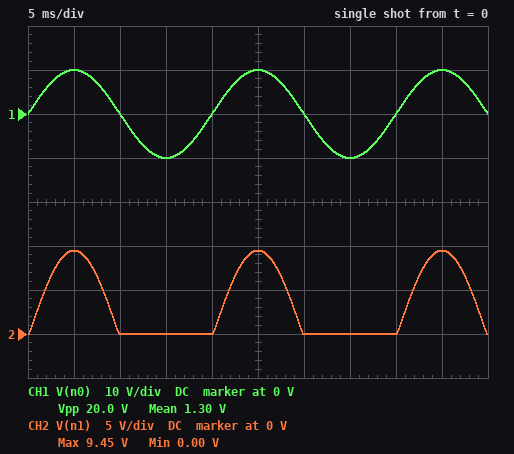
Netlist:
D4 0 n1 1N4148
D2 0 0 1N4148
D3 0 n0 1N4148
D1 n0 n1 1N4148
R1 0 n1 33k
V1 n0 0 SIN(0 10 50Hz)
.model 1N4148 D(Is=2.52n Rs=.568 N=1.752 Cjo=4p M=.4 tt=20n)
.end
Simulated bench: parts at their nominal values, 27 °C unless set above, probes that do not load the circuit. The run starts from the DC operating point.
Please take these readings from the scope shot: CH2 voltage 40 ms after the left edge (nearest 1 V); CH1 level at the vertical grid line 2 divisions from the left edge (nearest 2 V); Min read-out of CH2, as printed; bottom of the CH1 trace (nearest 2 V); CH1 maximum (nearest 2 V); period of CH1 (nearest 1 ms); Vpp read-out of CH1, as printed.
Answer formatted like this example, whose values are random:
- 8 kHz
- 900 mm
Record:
- 0 V
- 0 V
- 0.00 V
- -10 V
- 10 V
- 20 ms
- 20.0 V
